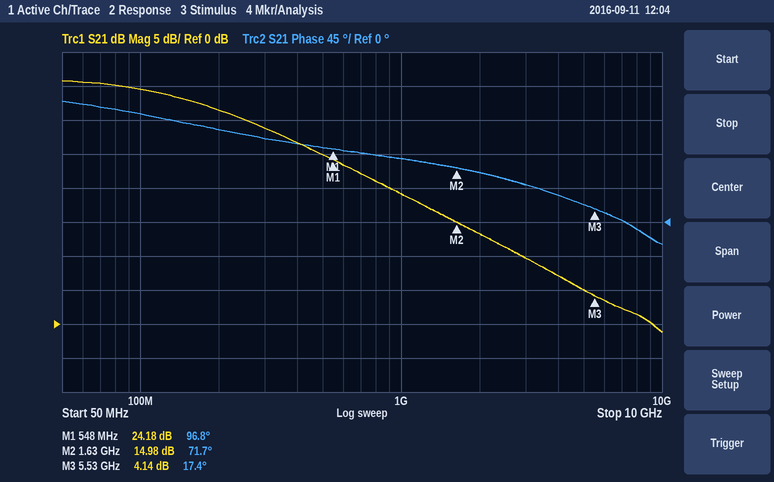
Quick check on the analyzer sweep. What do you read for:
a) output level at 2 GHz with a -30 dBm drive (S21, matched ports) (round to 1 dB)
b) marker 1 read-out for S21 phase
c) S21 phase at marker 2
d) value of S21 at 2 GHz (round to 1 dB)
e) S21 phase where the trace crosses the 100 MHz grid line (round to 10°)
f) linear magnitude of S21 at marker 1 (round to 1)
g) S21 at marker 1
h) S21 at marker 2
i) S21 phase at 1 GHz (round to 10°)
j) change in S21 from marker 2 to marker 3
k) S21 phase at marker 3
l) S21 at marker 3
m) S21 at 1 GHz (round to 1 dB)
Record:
-17 dBm
96.8°
71.7°
13 dB
140°
16
24.18 dB
14.98 dB
80°
-10.84 dB
17.4°
4.14 dB
19 dB
